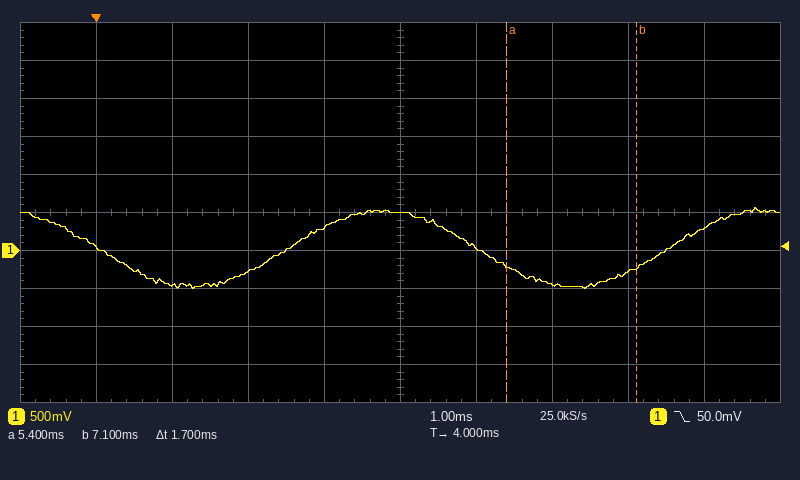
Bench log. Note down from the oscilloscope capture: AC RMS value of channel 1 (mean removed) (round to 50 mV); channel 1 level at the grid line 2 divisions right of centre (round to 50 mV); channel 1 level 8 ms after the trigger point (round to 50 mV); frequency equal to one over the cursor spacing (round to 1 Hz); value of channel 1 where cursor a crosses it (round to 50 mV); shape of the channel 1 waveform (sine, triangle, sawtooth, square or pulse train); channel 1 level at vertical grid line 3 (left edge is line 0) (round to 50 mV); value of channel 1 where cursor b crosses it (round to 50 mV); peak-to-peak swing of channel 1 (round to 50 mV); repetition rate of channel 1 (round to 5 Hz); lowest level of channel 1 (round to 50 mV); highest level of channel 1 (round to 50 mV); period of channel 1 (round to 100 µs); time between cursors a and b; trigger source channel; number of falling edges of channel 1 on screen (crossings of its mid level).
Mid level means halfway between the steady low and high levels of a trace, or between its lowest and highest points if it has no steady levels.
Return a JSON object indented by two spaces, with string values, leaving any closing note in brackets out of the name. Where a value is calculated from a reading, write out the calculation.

{
  "AC RMS value of channel 1 (mean removed)": "1.05 V / (2√2) ≈ 371 mV, so 350 mV to the nearest 50 mV",
  "channel 1 level at the grid line 2 divisions right of centre": "-450 mV",
  "channel 1 level 8 ms after the trigger point": "300 mV",
  "frequency equal to one over the cursor spacing": "1 / 1.7 ms ≈ 588 Hz",
  "value of channel 1 where cursor a crosses it": "-200 mV",
  "shape of the channel 1 waveform": "sine",
  "channel 1 level at vertical grid line 3 (left edge is line 0)": "-300 mV",
  "value of channel 1 where cursor b crosses it": "-200 mV",
  "peak-to-peak swing of channel 1": "550 mV − (-500 mV) = 1.05 V",
  "repetition rate of channel 1": "1 / 5.0 ms ≈ 200 Hz",
  "lowest level of channel 1": "-500 mV",
  "highest level of channel 1": "550 mV",
  "period of channel 1": "5.0 ms",
  "time between cursors a and b": "1.7 ms",
  "trigger source channel": "channel 1",
  "number of falling edges of channel 1 on screen": "2"
}
